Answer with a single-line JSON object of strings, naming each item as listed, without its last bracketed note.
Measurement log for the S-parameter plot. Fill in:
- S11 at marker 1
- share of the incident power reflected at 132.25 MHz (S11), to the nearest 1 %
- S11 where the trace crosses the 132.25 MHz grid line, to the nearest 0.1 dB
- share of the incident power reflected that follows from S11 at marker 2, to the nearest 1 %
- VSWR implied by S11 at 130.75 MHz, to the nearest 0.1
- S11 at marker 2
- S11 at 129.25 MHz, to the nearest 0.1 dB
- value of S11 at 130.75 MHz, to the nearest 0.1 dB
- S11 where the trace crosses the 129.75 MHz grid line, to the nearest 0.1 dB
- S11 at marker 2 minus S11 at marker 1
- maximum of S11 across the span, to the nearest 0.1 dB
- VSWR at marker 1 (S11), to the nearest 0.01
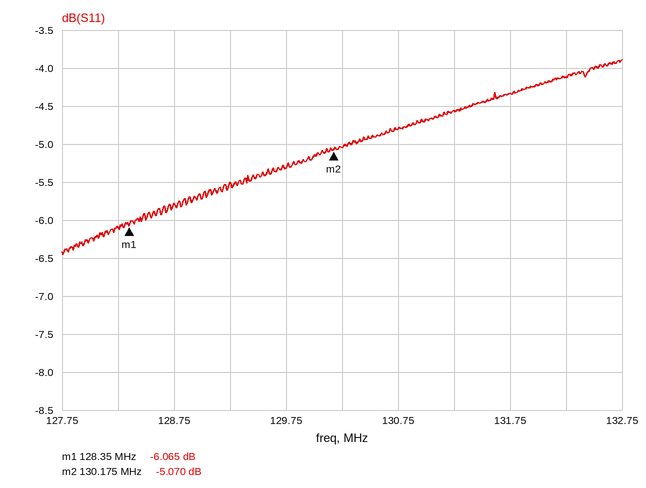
{"S11 at marker 1": "-6.065 dB", "share of the incident power reflected at 132.25 MHz (S11), to the nearest 1 %": "39 %", "S11 where the trace crosses the 132.25 MHz grid line, to the nearest 0.1 dB": "-4.1 dB", "share of the incident power reflected that follows from S11 at marker 2, to the nearest 1 %": "31 %", "VSWR implied by S11 at 130.75 MHz, to the nearest 0.1": "3.7", "S11 at marker 2": "-5.070 dB", "S11 at 129.25 MHz, to the nearest 0.1 dB": "-5.5 dB", "value of S11 at 130.75 MHz, to the nearest 0.1 dB": "-4.8 dB", "S11 where the trace crosses the 129.75 MHz grid line, to the nearest 0.1 dB": "-5.3 dB", "S11 at marker 2 minus S11 at marker 1": "0.995 dB", "maximum of S11 across the span, to the nearest 0.1 dB": "-3.9 dB", "VSWR at marker 1 (S11), to the nearest 0.01": "2.98"}
